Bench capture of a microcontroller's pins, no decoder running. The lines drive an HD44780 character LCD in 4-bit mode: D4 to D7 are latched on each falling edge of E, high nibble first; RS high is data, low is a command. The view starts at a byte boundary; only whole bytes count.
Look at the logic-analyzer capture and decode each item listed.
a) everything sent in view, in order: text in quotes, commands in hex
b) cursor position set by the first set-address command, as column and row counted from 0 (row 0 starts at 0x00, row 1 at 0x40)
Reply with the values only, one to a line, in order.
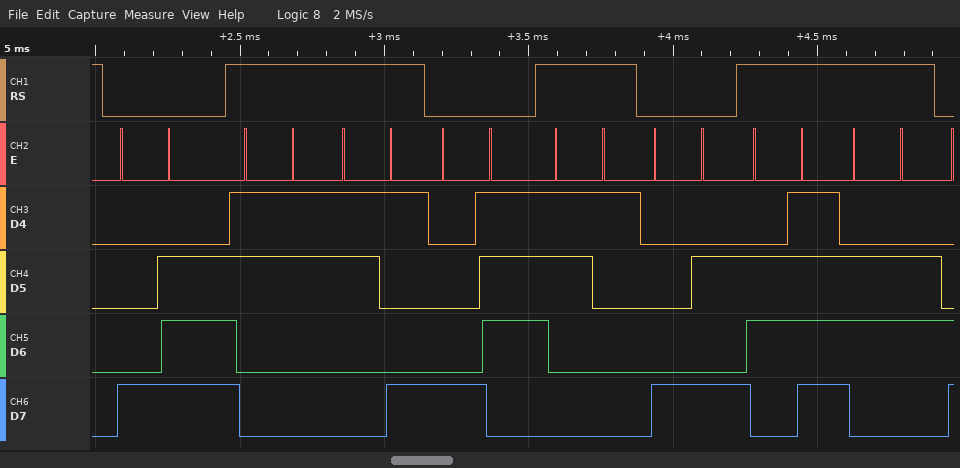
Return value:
0x8E "39" 0x87 "1" 0x8A "of"
column 14, row 0
